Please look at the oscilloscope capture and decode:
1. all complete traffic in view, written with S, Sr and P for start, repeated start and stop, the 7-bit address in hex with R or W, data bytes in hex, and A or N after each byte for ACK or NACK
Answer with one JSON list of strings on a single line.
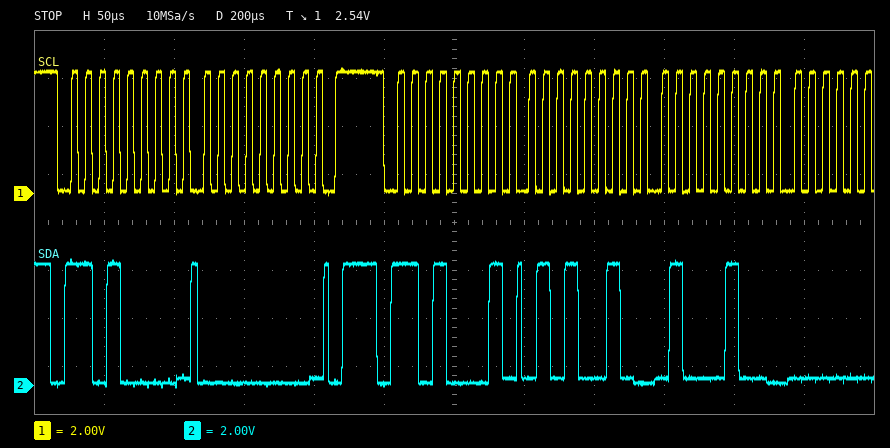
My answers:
["S 68W A 00 A P S 68R A 52 A 44 A"]
